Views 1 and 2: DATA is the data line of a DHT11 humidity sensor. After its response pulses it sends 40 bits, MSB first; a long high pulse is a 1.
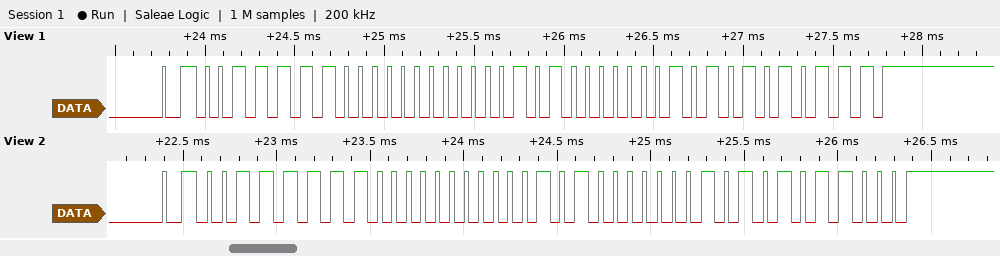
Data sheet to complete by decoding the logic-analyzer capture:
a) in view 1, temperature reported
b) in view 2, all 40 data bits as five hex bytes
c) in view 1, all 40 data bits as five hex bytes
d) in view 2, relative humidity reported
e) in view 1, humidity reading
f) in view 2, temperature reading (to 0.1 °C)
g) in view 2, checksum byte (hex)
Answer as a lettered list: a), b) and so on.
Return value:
a) 20.5 °C
b) 3F 00 14 05 58
c) 3E 00 14 05 57
d) 63 %
e) 62 %
f) 20.5 °C
g) 0x58
